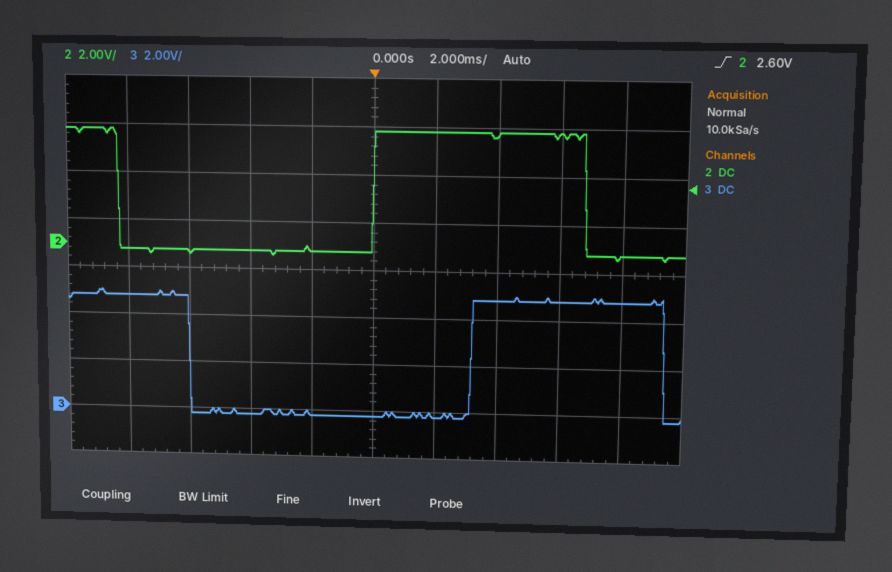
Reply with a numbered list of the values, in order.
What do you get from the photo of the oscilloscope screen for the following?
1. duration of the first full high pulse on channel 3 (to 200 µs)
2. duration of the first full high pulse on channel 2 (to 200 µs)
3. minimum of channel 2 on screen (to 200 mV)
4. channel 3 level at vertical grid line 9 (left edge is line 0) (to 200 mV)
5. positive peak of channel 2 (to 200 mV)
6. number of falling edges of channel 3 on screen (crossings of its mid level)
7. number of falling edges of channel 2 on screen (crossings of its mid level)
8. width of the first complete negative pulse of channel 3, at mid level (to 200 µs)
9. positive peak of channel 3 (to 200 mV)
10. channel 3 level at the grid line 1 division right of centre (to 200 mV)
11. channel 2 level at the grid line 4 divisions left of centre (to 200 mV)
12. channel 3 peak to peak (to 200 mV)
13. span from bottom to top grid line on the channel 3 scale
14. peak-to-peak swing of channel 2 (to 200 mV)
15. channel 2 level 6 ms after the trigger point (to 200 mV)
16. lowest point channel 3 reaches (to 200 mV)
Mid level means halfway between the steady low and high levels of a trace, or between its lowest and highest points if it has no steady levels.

1. 6.2 ms
2. 6.8 ms
3. -400 mV
4. 4.8 V
5. 4.8 V
6. 2
7. 2
8. 9.2 ms
9. 5.0 V
10. -200 mV
11. -200 mV
12. 5.2 V
13. 16 V
14. 5.2 V
15. 4.8 V
16. -200 mV
